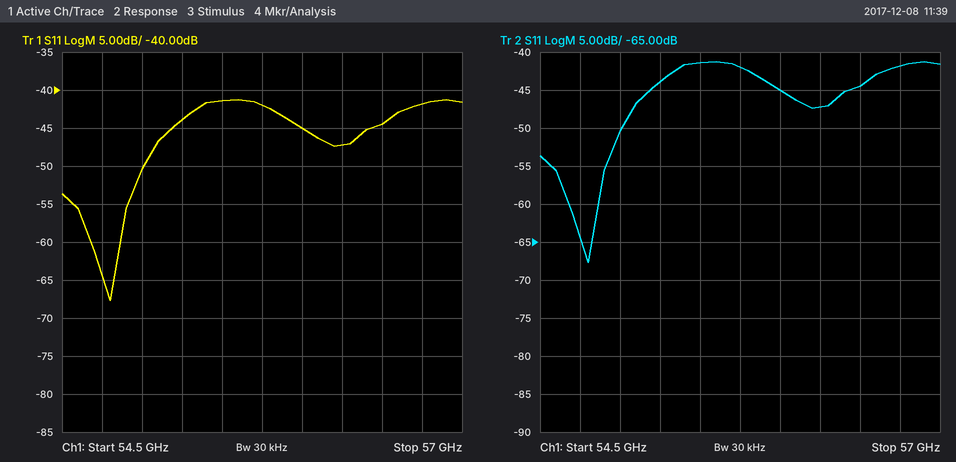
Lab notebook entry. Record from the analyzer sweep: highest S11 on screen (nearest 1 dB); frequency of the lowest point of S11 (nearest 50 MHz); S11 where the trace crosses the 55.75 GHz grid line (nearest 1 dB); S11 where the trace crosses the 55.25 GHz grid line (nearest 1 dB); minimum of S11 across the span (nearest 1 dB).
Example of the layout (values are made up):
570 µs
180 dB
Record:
-41 dB
54.80 GHz
-42 dB
-44 dB
-68 dB
